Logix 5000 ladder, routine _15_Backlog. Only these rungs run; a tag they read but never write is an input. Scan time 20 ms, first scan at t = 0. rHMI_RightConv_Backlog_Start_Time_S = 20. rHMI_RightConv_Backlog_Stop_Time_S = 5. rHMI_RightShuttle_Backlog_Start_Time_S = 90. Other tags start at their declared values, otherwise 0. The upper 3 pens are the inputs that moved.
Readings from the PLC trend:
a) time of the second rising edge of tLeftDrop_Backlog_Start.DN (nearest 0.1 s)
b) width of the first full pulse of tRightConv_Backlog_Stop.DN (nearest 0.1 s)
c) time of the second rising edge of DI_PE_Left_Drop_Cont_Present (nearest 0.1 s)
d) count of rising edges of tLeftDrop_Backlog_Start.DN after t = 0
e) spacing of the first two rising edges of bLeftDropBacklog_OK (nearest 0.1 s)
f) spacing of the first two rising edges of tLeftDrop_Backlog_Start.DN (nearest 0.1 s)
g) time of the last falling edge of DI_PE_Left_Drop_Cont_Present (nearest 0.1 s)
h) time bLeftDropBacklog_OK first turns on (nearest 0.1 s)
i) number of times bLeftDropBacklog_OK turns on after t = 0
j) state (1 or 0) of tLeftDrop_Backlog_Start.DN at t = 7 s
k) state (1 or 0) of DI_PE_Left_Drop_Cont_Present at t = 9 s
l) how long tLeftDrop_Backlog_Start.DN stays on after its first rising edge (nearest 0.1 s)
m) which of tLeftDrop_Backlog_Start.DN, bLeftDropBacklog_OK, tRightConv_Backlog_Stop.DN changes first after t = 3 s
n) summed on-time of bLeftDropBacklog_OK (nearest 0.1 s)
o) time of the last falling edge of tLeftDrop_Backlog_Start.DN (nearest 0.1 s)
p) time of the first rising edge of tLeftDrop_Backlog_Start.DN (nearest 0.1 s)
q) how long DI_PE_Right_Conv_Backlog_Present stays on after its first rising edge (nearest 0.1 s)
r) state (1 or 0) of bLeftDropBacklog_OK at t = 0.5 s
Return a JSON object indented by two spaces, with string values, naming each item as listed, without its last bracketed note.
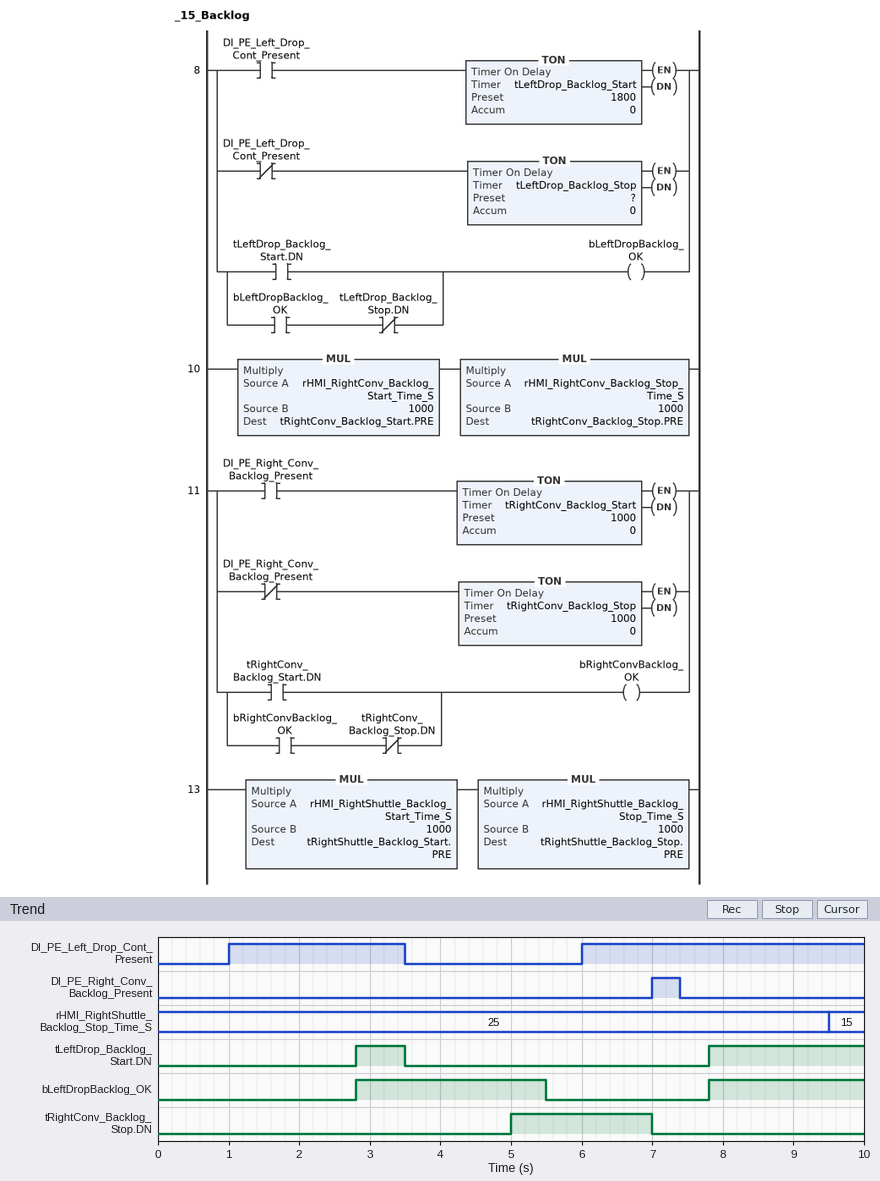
{
  "time of the second rising edge of tLeftDrop_Backlog_Start.DN": "7.8 s",
  "width of the first full pulse of tRightConv_Backlog_Stop.DN": "2.0 s",
  "time of the second rising edge of DI_PE_Left_Drop_Cont_Present": "6.0 s",
  "count of rising edges of tLeftDrop_Backlog_Start.DN after t = 0": "2",
  "spacing of the first two rising edges of bLeftDropBacklog_OK": "5.0 s",
  "spacing of the first two rising edges of tLeftDrop_Backlog_Start.DN": "5.0 s",
  "time of the last falling edge of DI_PE_Left_Drop_Cont_Present": "3.5 s",
  "time bLeftDropBacklog_OK first turns on": "2.8 s",
  "number of times bLeftDropBacklog_OK turns on after t = 0": "2",
  "state (1 or 0) of tLeftDrop_Backlog_Start.DN at t = 7 s": "0",
  "state (1 or 0) of DI_PE_Left_Drop_Cont_Present at t = 9 s": "1",
  "how long tLeftDrop_Backlog_Start.DN stays on after its first rising edge": "0.7 s",
  "which of tLeftDrop_Backlog_Start.DN, bLeftDropBacklog_OK, tRightConv_Backlog_Stop.DN changes first after t = 3 s": "tLeftDrop_Backlog_Start.DN",
  "summed on-time of bLeftDropBacklog_OK": "4.9 s",
  "time of the last falling edge of tLeftDrop_Backlog_Start.DN": "3.5 s",
  "time of the first rising edge of tLeftDrop_Backlog_Start.DN": "2.8 s",
  "how long DI_PE_Right_Conv_Backlog_Present stays on after its first rising edge": "0.4 s",
  "state (1 or 0) of bLeftDropBacklog_OK at t = 0.5 s": "0"
}
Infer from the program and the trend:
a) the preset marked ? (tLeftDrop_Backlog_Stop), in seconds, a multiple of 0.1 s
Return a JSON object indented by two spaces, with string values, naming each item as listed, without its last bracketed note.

{
  "the preset marked ? (tLeftDrop_Backlog_Stop), in seconds, a multiple of 0.1 s": "2.0 s"
}
